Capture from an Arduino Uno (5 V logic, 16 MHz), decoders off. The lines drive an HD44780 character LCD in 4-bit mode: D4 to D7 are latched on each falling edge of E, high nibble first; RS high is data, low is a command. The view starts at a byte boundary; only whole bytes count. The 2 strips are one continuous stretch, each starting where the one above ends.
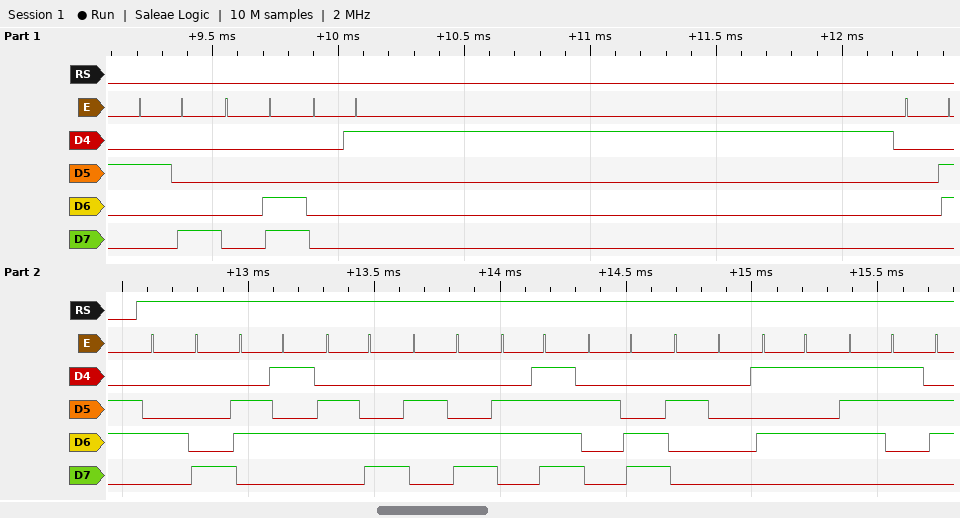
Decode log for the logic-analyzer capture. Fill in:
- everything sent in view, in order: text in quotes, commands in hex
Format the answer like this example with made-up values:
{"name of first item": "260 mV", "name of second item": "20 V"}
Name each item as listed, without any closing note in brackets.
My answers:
{"everything sent in view, in order: text in quotes, commands in hex": "0x28 0x0C 0x01 0x06 \"Hello, Us\""}
